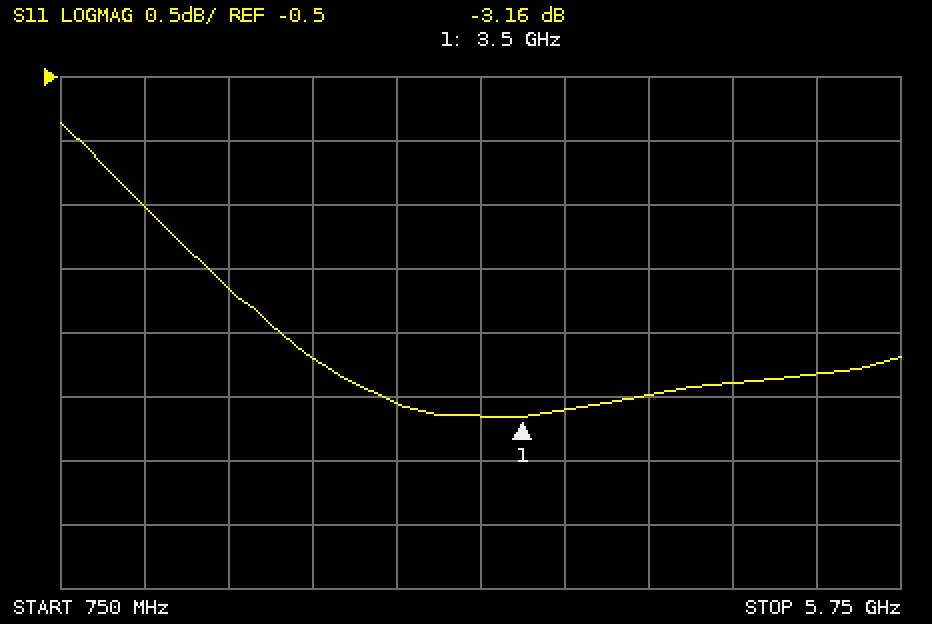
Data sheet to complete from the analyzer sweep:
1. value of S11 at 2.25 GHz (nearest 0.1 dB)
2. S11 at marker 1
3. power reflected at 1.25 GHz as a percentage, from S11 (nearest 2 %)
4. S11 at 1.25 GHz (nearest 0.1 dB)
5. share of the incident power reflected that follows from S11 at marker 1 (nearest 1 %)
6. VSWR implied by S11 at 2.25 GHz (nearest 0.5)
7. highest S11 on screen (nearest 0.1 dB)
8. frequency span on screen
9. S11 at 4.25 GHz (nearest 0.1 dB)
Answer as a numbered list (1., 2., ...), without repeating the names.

1. -2.7 dB
2. -3.16 dB
3. 70 %
4. -1.5 dB
5. 48 %
6. 6.5
7. -0.9 dB
8. 5 GHz
9. -3.0 dB
